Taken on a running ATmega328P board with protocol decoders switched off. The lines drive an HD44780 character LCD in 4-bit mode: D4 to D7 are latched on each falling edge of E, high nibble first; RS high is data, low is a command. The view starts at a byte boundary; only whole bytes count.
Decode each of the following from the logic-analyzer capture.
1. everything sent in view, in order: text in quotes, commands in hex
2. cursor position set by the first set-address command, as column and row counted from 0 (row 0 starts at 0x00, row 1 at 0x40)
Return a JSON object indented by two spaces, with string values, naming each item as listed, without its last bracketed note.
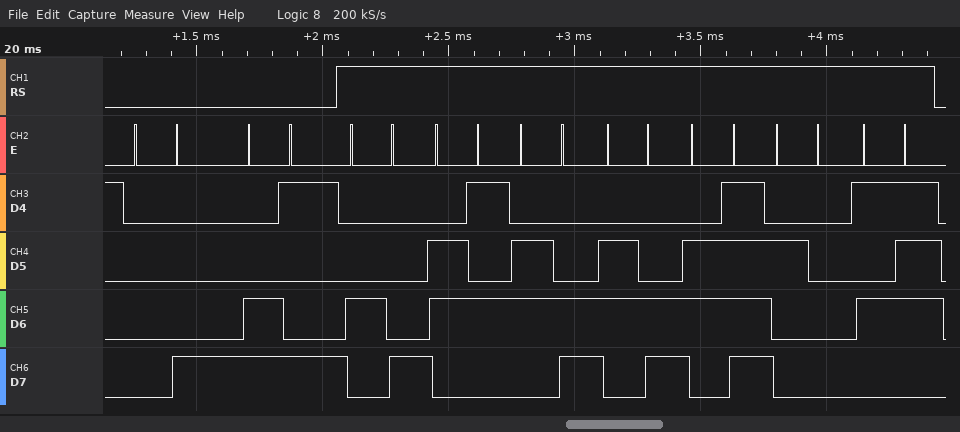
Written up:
{
  "everything sent in view, in order: text in quotes, commands in hex": "0x08 0xC9 \"Hello W\"",
  "cursor position set by the first set-address command, as column and row counted from 0": "column 9, row 1"
}
